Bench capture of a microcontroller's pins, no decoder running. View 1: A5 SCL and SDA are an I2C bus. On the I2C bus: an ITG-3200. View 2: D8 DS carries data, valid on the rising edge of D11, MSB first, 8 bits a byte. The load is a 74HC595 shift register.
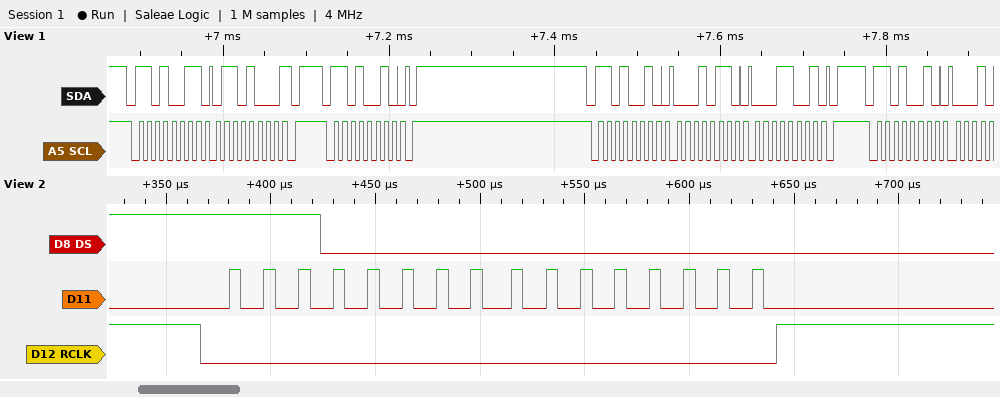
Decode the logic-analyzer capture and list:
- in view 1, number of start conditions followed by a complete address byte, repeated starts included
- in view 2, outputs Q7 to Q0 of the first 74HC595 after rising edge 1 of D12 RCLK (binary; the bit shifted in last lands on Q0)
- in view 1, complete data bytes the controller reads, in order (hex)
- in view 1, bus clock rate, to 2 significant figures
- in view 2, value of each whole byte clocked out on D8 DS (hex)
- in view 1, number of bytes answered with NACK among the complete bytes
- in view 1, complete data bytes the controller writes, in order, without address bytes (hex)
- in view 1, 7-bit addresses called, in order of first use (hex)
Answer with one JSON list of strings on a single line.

["4", "00000000", "68", "100 kHz", "E0 00", "1", "16 19", "0x69"]
